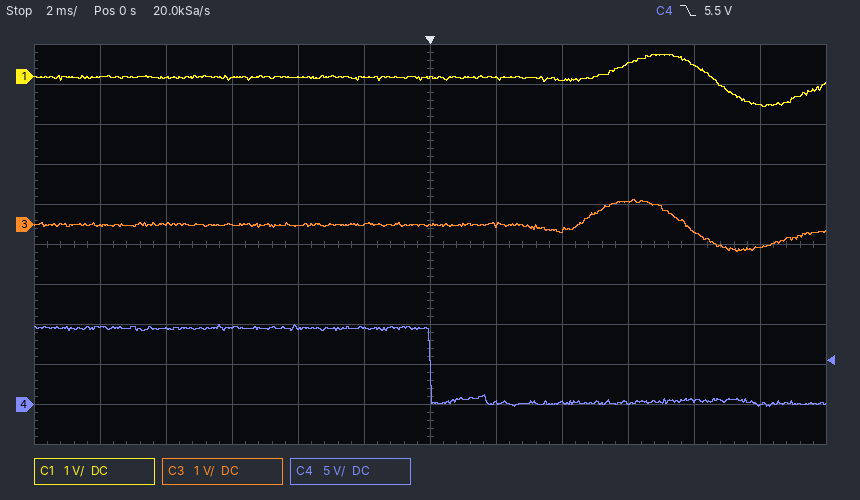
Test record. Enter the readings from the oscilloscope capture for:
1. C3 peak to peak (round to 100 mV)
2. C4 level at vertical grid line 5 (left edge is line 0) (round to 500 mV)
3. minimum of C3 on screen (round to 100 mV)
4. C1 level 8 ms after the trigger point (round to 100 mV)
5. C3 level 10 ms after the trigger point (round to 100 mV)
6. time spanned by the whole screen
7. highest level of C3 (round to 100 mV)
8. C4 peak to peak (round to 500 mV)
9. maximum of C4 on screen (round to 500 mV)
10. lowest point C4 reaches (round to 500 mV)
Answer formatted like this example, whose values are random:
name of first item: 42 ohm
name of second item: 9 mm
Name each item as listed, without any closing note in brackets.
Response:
C3 peak to peak: 1.3 V
C4 level at vertical grid line 5 (left edge is line 0): 9.5 V
minimum of C3 on screen: -700 mV
C1 level 8 ms after the trigger point: 300 mV
C3 level 10 ms after the trigger point: -600 mV
time spanned by the whole screen: 24 ms
highest level of C3: 600 mV
C4 peak to peak: 10.0 V
maximum of C4 on screen: 10.0 V
lowest point C4 reaches: 0.0 V
